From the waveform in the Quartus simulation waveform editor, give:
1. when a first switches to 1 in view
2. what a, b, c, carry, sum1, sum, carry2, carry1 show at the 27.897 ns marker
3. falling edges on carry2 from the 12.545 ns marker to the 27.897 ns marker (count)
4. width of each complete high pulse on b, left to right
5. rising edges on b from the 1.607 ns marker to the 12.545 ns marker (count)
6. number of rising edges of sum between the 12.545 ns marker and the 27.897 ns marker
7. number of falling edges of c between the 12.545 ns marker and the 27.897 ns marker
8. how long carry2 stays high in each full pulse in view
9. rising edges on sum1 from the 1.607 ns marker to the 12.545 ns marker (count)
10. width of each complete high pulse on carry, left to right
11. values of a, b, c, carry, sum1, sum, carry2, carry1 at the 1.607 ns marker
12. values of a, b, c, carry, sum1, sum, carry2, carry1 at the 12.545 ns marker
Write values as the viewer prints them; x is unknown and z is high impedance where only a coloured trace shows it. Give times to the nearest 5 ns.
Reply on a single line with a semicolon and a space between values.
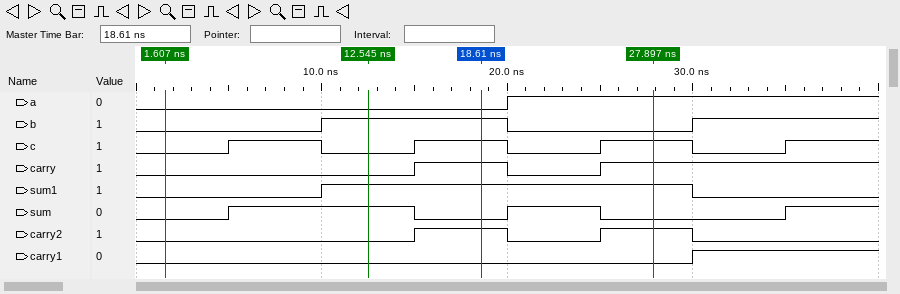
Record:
20 ns; a=1, b=0, c=1, carry=1, sum1=1, sum=0, carry2=1, carry1=0; 1; 10 ns; 1; 1; 1; 5 ns, 5 ns; 1; 5 ns; a=0, b=0, c=0, carry=0, sum1=0, sum=0, carry2=0, carry1=0; a=0, b=1, c=0, carry=0, sum1=1, sum=1, carry2=0, carry1=0
